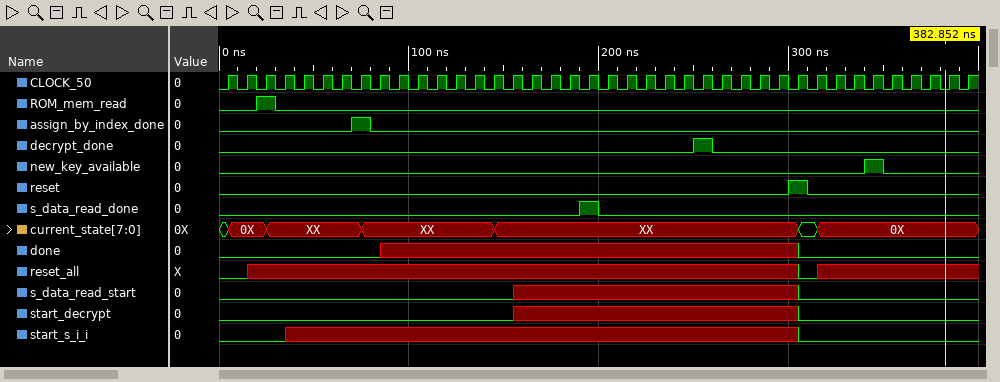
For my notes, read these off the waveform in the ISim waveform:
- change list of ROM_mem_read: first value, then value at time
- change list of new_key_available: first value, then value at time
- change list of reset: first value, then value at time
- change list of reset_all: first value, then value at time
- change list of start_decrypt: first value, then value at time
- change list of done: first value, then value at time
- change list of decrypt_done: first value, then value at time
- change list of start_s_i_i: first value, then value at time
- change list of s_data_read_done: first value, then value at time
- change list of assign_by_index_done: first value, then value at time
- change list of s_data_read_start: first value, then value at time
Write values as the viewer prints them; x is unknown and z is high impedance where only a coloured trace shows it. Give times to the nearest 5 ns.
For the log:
0, 1 at 20 ns, 0 at 30 ns
0, 1 at 340 ns, 0 at 350 ns
0, 1 at 300 ns, 0 at 310 ns
0, x at 15 ns, 0 at 305 ns, x at 315 ns
0, x at 155 ns, 0 at 305 ns
0, x at 85 ns, 0 at 305 ns
0, 1 at 250 ns, 0 at 260 ns
0, x at 35 ns, 0 at 305 ns
0, 1 at 190 ns, 0 at 200 ns
0, 1 at 70 ns, 0 at 80 ns
0, x at 155 ns, 0 at 305 ns
